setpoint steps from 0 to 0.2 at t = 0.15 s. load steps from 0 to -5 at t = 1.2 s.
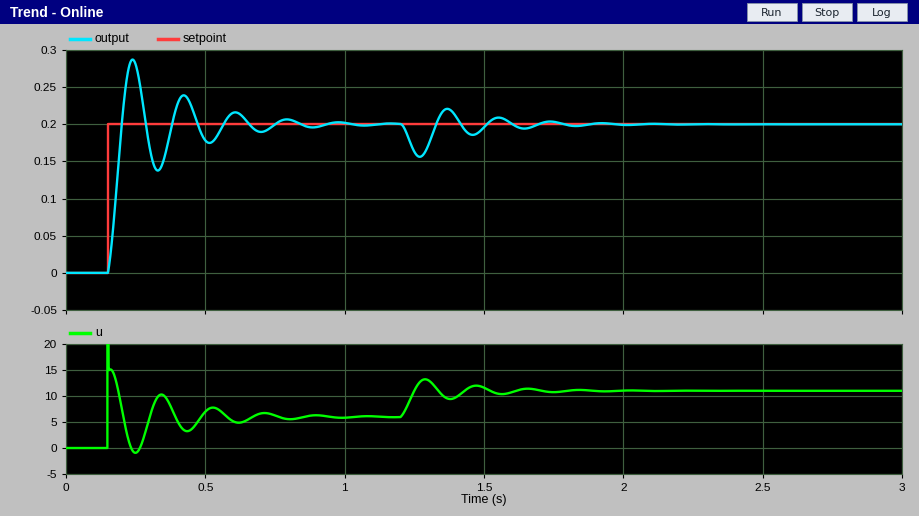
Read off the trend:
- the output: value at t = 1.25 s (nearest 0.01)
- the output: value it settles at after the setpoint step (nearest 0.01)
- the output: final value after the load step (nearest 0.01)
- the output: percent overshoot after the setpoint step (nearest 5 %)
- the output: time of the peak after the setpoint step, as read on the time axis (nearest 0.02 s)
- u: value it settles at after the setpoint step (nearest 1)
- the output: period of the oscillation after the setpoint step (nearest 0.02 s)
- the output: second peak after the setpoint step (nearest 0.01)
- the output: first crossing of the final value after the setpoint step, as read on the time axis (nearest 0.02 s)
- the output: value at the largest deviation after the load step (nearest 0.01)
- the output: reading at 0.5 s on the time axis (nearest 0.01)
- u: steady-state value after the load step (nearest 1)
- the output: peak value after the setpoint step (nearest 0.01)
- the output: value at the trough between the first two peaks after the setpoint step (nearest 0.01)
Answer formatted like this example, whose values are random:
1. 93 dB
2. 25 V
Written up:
1. 0.16
2. 0.20
3. 0.20
4. 45 %
5. 0.24 s
6. 6
7. 0.18 s
8. 0.24
9. 0.20 s
10. 0.16
11. 0.18
12. 11
13. 0.29
14. 0.14
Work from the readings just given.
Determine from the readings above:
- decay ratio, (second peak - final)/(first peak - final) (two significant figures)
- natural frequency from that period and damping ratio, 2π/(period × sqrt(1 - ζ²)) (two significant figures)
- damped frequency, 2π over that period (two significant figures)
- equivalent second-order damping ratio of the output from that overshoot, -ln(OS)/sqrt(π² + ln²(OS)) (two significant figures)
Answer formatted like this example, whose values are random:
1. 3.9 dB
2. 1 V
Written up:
1. 0.44
2. 36 rad/s
3. 35 rad/s
4. 0.25
